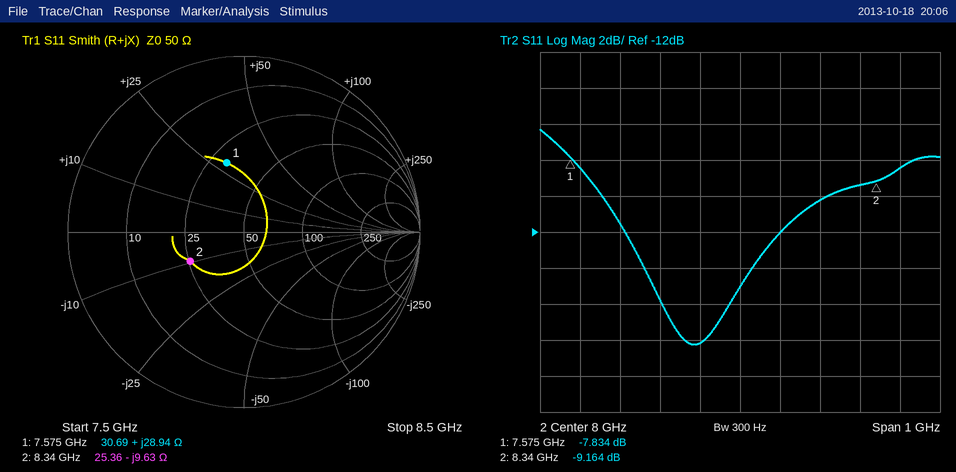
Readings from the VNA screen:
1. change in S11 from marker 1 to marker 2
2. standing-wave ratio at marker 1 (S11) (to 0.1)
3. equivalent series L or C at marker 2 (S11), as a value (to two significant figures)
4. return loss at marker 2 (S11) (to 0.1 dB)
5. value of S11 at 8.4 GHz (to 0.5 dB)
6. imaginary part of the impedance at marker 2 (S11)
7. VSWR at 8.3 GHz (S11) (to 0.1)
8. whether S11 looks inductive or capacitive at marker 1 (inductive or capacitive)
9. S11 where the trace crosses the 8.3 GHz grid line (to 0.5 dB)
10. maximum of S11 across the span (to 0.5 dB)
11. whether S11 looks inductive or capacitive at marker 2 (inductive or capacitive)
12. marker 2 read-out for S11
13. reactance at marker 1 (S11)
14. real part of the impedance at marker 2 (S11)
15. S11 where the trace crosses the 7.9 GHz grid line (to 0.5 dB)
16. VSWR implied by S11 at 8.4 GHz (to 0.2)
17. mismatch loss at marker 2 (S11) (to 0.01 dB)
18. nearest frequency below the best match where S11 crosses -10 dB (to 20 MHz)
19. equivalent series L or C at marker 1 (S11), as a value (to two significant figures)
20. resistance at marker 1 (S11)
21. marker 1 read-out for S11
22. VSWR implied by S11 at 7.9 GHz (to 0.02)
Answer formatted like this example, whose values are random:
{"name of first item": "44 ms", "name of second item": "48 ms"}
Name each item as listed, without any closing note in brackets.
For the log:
{"change in S11 from marker 1 to marker 2": "-1.330 dB", "standing-wave ratio at marker 1 (S11)": "2.4", "equivalent series L or C at marker 2 (S11), as a value": "2.0 pF", "return loss at marker 2 (S11)": "9.2 dB", "value of S11 at 8.4 GHz": "-8.5 dB", "imaginary part of the impedance at marker 2": "-9.63 Ω", "VSWR at 8.3 GHz (S11)": "2.0", "whether S11 looks inductive or capacitive at marker 1": "inductive", "S11 where the trace crosses the 8.3 GHz grid line": "-9.5 dB", "maximum of S11 across the span": "-6.5 dB", "whether S11 looks inductive or capacitive at marker 2": "capacitive", "marker 2 read-out for S11": "-9.164 dB", "reactance at marker 1": "+28.94 Ω", "real part of the impedance at marker 2": "25.36 Ω", "S11 where the trace crosses the 7.9 GHz grid line": "-18.0 dB", "VSWR implied by S11 at 8.4 GHz": "2.2", "mismatch loss at marker 2 (S11)": "0.56 dB", "nearest frequency below the best match where S11 crosses -10 dB": "7.66 GHz", "equivalent series L or C at marker 1 (S11), as a value": "610 pH", "resistance at marker 1": "30.69 Ω", "marker 1 read-out for S11": "-7.834 dB", "VSWR implied by S11 at 7.9 GHz": "1.28"}
